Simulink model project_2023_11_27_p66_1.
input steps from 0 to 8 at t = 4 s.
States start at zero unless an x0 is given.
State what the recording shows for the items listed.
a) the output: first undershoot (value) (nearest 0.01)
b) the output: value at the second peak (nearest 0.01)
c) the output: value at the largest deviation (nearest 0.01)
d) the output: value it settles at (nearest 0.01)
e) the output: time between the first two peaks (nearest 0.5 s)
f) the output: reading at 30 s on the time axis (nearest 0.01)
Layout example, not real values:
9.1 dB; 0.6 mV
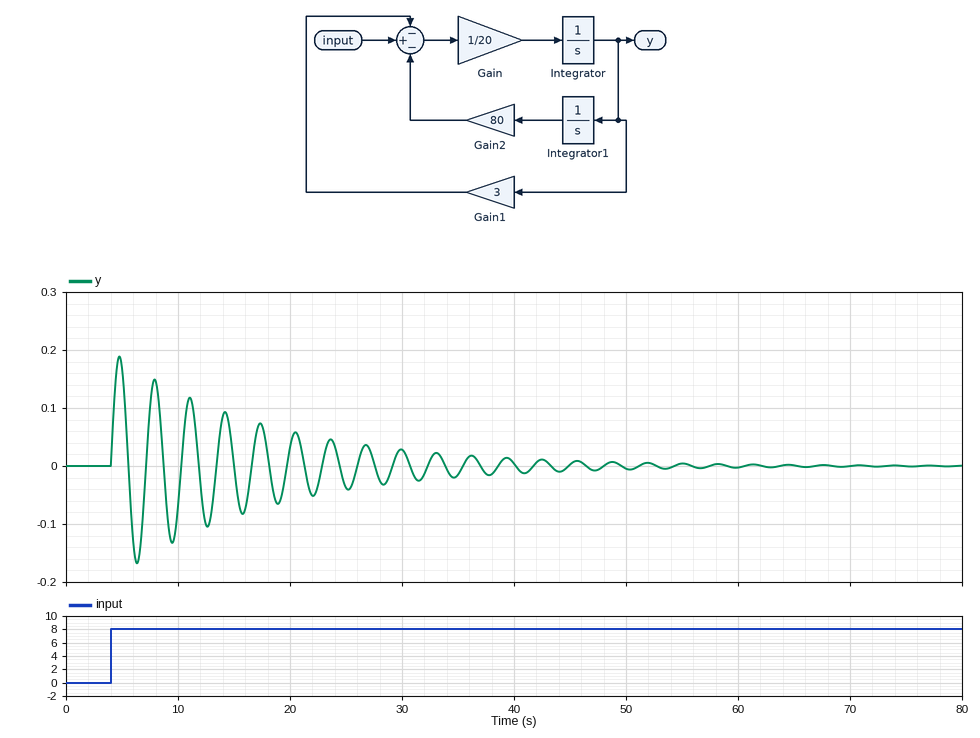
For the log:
-0.17; 0.15; 0.19; 0.00; 3.0 s; 0.03
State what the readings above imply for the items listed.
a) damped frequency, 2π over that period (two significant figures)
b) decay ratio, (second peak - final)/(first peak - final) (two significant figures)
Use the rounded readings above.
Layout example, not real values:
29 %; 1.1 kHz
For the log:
2.1 rad/s; 0.79
